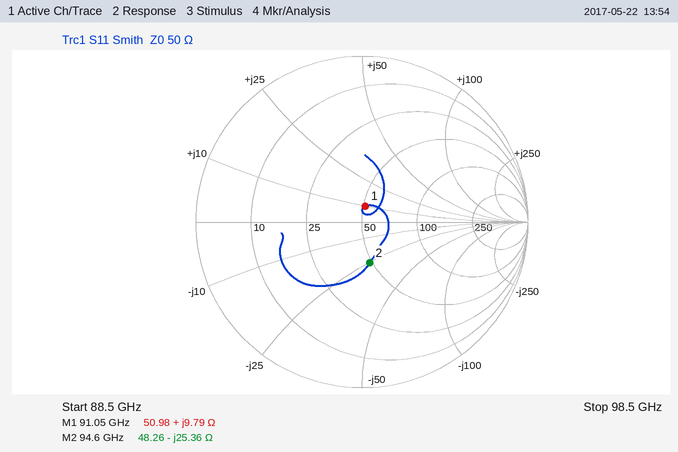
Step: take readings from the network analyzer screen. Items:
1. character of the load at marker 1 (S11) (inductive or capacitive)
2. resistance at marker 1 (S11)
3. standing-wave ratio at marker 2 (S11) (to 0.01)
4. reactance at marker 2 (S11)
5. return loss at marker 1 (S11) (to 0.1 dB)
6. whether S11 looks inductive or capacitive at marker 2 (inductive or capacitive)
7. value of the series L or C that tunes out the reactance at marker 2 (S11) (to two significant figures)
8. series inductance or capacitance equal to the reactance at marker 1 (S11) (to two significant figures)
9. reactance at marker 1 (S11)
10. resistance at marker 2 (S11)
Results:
inductive
50.98 Ω
1.67
-25.36 Ω
20.3 dB
capacitive
43 pH
17 pH
+9.79 Ω
48.26 Ω
